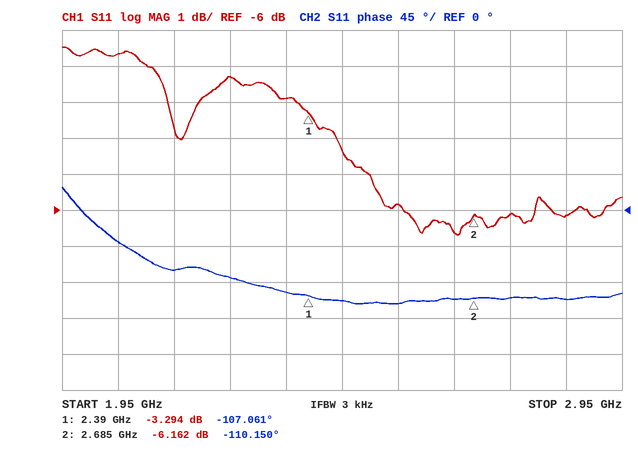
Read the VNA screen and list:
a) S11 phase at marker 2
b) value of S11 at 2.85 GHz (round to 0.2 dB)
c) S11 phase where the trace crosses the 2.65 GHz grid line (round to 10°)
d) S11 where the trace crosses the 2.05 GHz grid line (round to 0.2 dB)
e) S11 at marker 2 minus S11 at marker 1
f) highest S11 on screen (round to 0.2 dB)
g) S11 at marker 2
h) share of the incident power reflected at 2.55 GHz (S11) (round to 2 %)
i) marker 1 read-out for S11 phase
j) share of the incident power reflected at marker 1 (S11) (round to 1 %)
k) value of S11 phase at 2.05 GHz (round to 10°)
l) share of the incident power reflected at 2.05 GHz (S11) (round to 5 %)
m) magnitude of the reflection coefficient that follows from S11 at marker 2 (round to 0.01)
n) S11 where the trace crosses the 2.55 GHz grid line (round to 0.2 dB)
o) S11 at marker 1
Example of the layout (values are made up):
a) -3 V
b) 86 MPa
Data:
a) -110.150°
b) -6.2 dB
c) -110°
d) -1.6 dB
e) -2.868 dB
f) -1.4 dB
g) -6.162 dB
h) 26 %
i) -107.061°
j) 47 %
k) -40°
l) 70 %
m) 0.49
n) -5.8 dB
o) -3.294 dB
